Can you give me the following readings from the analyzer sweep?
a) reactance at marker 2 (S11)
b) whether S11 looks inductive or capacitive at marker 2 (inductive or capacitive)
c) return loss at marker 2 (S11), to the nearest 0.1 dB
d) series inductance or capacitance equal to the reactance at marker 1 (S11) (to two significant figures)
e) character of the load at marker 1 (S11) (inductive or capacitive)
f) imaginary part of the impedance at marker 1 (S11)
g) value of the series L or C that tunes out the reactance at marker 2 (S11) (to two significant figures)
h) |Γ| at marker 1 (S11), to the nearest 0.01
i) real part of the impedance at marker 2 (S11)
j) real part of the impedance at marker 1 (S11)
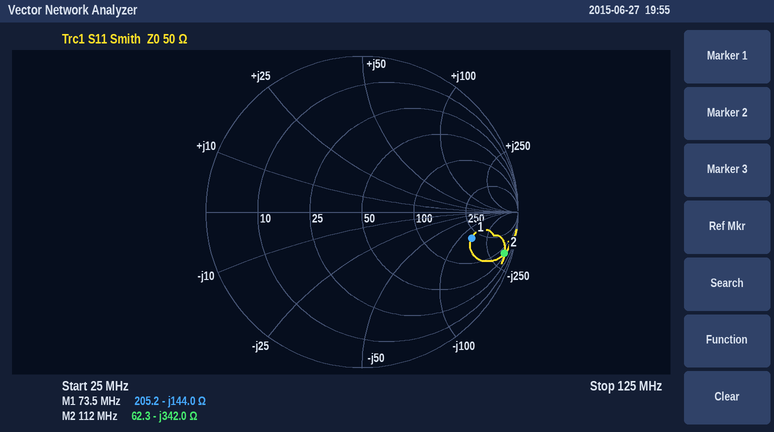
-342.0 Ω
capacitive
0.4 dB
15 pF
capacitive
-144.0 Ω
490 nH
0.72
62.3 Ω
205.2 Ω
